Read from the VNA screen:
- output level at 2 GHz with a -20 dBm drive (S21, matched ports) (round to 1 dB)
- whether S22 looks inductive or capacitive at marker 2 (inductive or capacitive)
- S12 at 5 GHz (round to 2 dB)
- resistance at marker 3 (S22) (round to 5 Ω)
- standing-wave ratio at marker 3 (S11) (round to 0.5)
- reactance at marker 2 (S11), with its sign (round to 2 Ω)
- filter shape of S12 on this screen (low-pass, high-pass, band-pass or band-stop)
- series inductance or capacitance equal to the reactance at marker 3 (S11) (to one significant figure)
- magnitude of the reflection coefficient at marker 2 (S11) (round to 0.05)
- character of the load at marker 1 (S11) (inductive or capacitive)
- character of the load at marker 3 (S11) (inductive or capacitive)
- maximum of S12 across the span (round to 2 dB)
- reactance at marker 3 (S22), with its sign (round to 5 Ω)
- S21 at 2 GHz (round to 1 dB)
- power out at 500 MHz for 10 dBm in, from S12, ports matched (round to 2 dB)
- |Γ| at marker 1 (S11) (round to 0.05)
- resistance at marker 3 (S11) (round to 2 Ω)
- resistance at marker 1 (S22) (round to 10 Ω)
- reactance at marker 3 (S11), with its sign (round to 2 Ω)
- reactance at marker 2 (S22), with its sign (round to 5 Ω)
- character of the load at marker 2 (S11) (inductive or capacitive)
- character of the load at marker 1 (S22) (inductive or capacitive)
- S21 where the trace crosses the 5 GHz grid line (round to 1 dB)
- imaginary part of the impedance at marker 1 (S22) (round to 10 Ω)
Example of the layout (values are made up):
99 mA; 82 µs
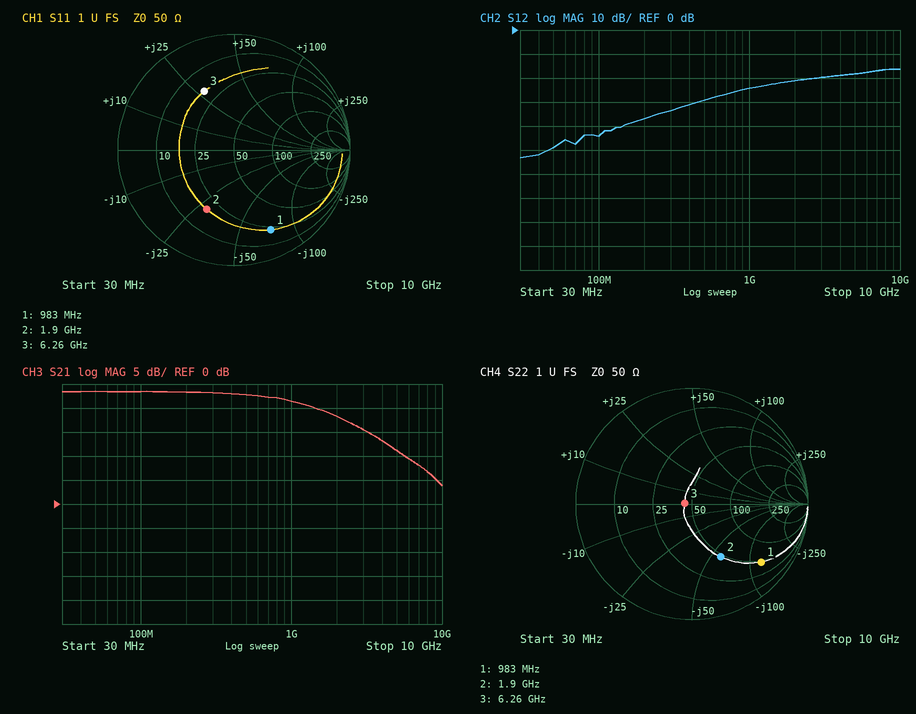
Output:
-2 dBm; capacitive; -18 dB; 45 Ω; 3.5; -28 Ω; high-pass; 700 pH; 0.55; capacitive; inductive; -16 dB; 0 Ω; 18 dB; -20 dBm; 0.75; 18 Ω; 50 Ω; +28 Ω; -60 Ω; capacitive; capacitive; 11 dB; -120 Ω
